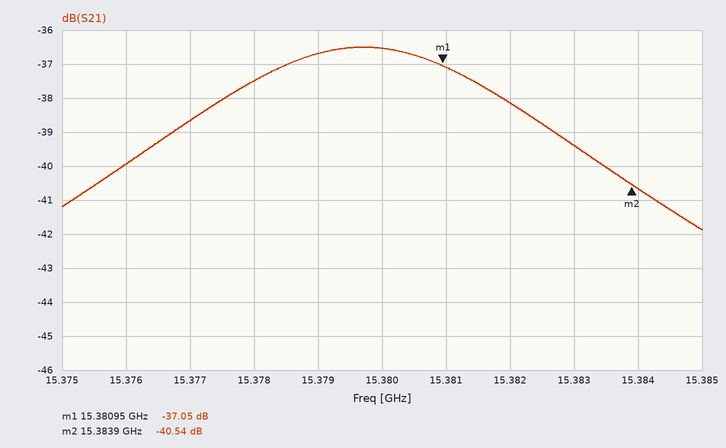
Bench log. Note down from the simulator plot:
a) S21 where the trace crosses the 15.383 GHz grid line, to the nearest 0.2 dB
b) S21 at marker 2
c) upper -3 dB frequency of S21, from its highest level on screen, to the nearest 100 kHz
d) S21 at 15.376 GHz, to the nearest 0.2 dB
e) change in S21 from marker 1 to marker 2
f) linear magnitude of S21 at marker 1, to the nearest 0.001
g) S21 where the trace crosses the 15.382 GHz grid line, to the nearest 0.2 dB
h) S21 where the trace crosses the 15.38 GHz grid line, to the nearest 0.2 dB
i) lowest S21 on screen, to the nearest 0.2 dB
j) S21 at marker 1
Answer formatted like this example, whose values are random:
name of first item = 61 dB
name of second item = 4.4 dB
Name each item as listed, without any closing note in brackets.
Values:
S21 where the trace crosses the 15.383 GHz grid line, to the nearest 0.2 dB = -39.4 dB
S21 at marker 2 = -40.54 dB
upper -3 dB frequency of S21, from its highest level on screen, to the nearest 100 kHz = 15.3831 GHz
S21 at 15.376 GHz, to the nearest 0.2 dB = -40.0 dB
change in S21 from marker 1 to marker 2 = -3.49 dB
linear magnitude of S21 at marker 1, to the nearest 0.001 = 0.014
S21 where the trace crosses the 15.382 GHz grid line, to the nearest 0.2 dB = -38.2 dB
S21 where the trace crosses the 15.38 GHz grid line, to the nearest 0.2 dB = -36.6 dB
lowest S21 on screen, to the nearest 0.2 dB = -41.8 dB
S21 at marker 1 = -37.05 dB
